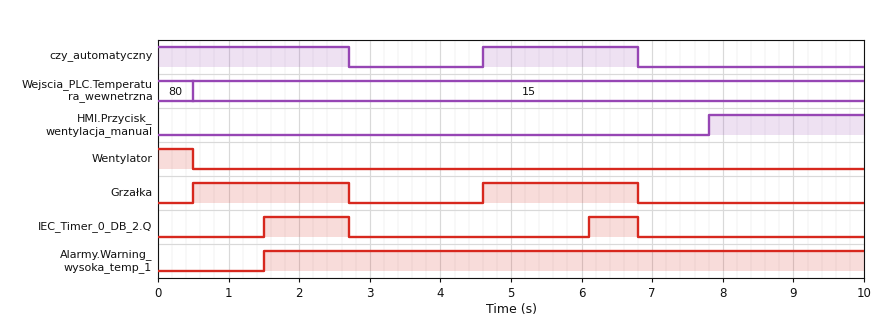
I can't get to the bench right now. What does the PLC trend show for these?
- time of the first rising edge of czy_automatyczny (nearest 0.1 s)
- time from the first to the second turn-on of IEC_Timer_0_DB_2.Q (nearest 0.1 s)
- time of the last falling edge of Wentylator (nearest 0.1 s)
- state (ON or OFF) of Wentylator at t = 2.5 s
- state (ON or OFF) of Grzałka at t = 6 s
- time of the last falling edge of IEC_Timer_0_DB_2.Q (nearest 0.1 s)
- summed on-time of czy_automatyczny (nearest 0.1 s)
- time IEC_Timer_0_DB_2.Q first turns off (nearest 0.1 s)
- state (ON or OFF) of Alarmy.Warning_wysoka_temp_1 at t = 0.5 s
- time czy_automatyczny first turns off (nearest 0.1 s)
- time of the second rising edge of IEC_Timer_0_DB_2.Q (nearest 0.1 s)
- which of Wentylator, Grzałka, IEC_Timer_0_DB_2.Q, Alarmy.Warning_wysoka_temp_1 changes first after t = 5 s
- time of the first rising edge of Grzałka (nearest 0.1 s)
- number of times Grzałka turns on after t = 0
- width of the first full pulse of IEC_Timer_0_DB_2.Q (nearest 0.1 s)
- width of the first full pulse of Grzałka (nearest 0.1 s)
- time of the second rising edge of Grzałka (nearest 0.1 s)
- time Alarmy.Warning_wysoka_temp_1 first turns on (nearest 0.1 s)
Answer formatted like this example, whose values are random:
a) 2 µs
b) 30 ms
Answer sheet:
a) 4.6 s
b) 4.6 s
c) 0.5 s
d) OFF
e) ON
f) 6.8 s
g) 4.9 s
h) 2.7 s
i) OFF
j) 2.7 s
k) 6.1 s
l) IEC_Timer_0_DB_2.Q
m) 0.5 s
n) 2
o) 1.2 s
p) 2.2 s
q) 4.6 s
r) 1.5 s
